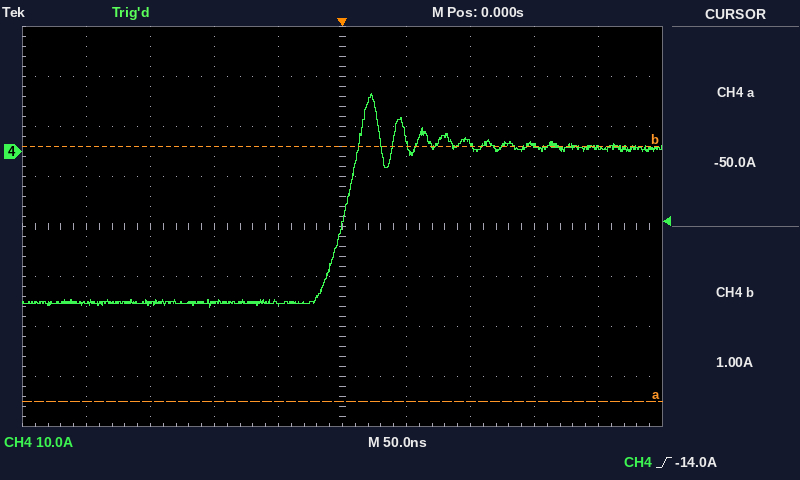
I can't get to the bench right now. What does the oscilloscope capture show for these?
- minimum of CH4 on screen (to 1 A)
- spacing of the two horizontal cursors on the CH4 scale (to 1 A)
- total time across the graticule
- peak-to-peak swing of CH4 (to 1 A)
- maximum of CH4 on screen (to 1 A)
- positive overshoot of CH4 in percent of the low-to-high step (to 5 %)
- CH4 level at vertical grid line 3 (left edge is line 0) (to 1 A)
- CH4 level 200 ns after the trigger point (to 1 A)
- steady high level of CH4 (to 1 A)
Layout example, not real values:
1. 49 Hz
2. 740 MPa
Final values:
1. -31 A
2. 51 A
3. 500 ns
4. 43 A
5. 12 A
6. 35 %
7. -30 A
8. 1 A
9. 1 A
